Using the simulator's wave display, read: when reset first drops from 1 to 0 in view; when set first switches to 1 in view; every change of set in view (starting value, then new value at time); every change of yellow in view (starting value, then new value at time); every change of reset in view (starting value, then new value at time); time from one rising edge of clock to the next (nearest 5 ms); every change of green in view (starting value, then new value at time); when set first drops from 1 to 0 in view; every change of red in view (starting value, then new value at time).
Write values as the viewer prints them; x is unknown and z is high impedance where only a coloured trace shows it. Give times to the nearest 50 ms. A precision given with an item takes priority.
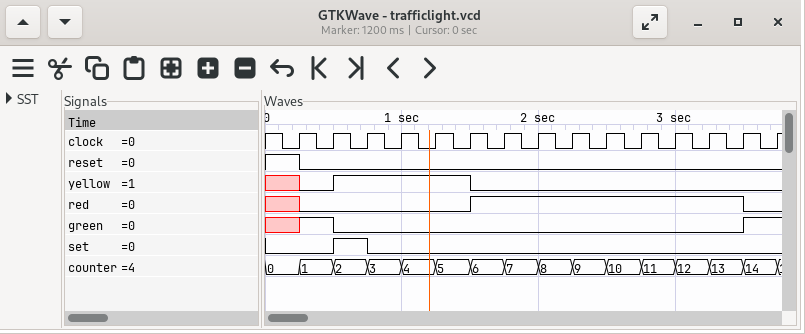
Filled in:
250 ms
500 ms
0, 1 at 500 ms, 0 at 750 ms
x, 0 at 250 ms, 1 at 500 ms, 0 at 1500 ms
1, 0 at 250 ms
250 ms
x, 1 at 250 ms, 0 at 500 ms, 1 at 3500 ms
750 ms
x, 0 at 250 ms, 1 at 1500 ms, 0 at 3500 ms
